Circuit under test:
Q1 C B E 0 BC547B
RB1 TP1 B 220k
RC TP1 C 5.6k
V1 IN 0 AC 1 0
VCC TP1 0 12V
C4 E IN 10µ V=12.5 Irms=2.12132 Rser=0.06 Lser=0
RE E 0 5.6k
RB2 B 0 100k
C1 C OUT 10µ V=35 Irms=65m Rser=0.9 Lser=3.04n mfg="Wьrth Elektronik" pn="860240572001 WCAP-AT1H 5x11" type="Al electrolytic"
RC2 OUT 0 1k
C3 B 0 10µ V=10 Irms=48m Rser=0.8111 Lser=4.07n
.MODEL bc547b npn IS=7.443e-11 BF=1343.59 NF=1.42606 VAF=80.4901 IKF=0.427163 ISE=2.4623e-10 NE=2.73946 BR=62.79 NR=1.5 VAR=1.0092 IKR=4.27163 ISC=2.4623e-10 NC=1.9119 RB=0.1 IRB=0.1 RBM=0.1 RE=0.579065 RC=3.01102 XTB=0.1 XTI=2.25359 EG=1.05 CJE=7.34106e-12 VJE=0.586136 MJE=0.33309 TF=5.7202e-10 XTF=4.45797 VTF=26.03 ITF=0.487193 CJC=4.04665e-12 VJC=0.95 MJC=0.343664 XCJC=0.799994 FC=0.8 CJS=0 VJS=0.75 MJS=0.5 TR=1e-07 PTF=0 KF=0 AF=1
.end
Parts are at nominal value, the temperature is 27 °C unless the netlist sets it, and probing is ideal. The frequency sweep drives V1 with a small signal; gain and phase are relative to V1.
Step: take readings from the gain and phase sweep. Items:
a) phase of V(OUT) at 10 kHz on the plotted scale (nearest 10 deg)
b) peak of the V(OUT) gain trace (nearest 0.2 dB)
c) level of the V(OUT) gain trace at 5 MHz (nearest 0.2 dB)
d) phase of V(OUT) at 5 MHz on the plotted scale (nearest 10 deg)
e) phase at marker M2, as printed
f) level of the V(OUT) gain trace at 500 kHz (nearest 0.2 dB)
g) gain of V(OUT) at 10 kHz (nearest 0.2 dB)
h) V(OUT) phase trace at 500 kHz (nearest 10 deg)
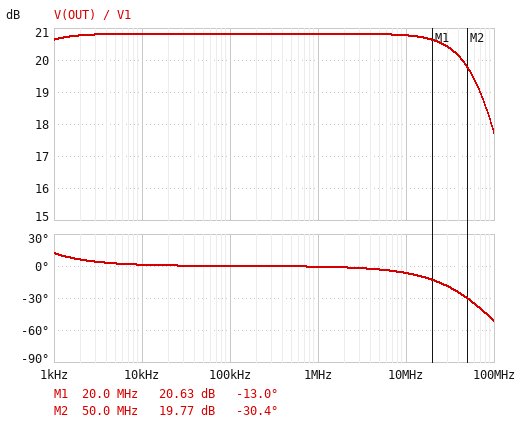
0 deg
20.8 dB
20.8 dB
0 deg
-30.4 deg
20.8 dB
20.8 dB
0 deg
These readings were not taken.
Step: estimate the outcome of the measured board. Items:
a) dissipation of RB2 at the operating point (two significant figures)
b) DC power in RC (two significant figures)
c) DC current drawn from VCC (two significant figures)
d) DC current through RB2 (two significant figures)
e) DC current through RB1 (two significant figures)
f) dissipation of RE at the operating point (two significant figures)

130 µW
1.6 mW
570 µA
36 µA
38 µA
1.6 mW
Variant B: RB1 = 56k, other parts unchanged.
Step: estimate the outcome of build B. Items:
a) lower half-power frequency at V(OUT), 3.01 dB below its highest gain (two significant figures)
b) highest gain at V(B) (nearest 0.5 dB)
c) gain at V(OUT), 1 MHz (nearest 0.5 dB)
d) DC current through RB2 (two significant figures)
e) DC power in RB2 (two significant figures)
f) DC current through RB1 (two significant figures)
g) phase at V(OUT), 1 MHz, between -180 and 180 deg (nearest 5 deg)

310 Hz
7.5 dB
17.0 dB
67 µA
450 µW
95 µA
-40 deg
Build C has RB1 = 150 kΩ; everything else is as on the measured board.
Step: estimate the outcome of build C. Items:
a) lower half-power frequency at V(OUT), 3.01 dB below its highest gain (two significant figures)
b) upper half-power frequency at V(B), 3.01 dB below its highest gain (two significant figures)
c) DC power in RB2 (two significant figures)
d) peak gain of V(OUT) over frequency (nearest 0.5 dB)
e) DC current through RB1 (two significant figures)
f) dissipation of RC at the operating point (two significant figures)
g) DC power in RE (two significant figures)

280 Hz
600 MHz
210 µW
23.0 dB
49 µA
2.8 mW
2.9 mW
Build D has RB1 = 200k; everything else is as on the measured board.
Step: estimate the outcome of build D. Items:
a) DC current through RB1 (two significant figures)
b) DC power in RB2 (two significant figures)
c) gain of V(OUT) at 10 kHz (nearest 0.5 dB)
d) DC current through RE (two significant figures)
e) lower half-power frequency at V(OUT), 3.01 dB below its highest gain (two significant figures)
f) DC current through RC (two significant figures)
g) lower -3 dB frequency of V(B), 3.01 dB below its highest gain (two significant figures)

41 µA
150 µW
21.5 dB
580 µA
230 Hz
570 µA
430 MHz
